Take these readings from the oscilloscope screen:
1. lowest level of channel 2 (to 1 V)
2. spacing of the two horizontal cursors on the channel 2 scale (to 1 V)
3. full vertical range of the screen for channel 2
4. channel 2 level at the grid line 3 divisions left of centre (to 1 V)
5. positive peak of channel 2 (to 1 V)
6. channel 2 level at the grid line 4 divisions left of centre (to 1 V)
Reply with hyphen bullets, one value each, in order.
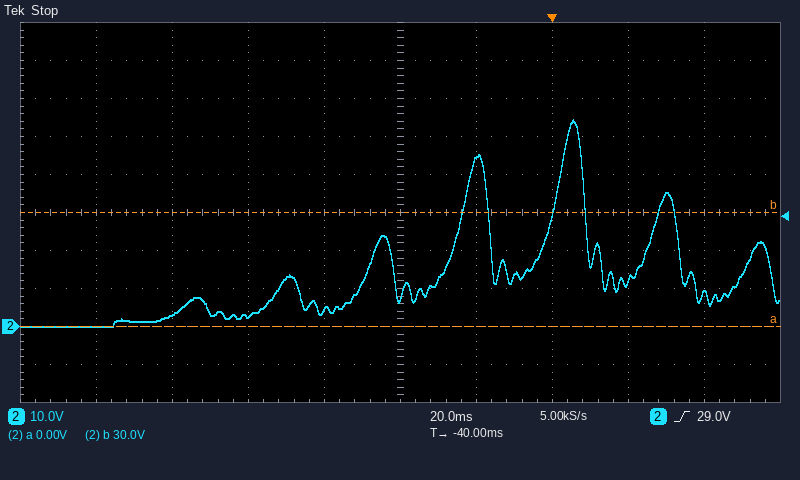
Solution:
- 0 V
- 30 V
- 100 V
- 3 V
- 54 V
- 0 V
